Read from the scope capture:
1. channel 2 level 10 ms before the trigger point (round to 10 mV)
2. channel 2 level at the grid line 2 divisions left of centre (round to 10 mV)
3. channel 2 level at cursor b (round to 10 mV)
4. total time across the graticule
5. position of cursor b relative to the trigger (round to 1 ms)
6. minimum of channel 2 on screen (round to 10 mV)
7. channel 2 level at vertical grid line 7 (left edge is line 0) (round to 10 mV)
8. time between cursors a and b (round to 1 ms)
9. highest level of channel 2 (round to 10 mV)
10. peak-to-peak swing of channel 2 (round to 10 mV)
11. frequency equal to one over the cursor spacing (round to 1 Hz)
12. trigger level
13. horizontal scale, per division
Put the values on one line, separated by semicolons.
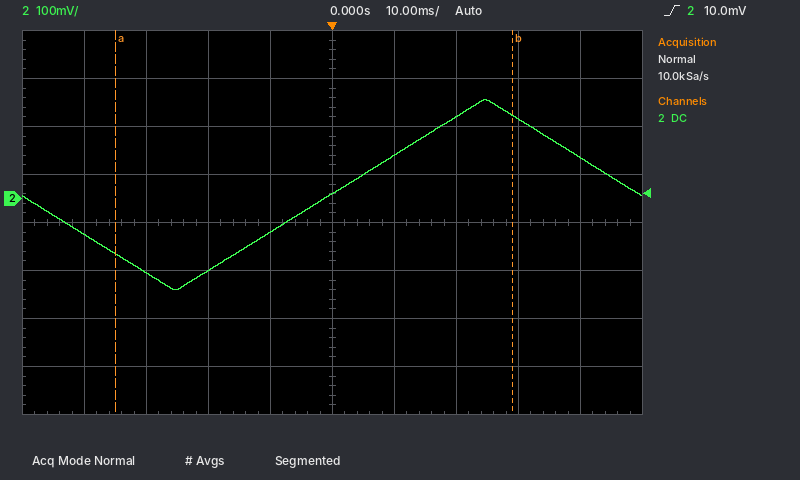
-70 mV; -150 mV; 170 mV; 100 ms; +29 ms; -190 mV; 170 mV; 64 ms; 210 mV; 400 mV; 16 Hz; 10.0 mV; 10 ms
